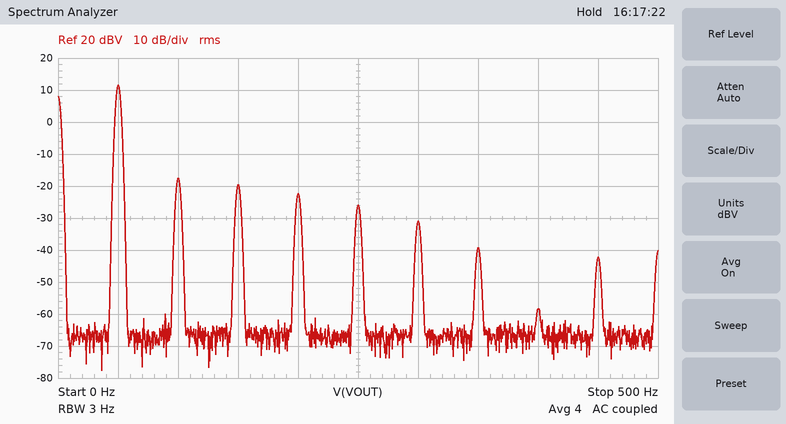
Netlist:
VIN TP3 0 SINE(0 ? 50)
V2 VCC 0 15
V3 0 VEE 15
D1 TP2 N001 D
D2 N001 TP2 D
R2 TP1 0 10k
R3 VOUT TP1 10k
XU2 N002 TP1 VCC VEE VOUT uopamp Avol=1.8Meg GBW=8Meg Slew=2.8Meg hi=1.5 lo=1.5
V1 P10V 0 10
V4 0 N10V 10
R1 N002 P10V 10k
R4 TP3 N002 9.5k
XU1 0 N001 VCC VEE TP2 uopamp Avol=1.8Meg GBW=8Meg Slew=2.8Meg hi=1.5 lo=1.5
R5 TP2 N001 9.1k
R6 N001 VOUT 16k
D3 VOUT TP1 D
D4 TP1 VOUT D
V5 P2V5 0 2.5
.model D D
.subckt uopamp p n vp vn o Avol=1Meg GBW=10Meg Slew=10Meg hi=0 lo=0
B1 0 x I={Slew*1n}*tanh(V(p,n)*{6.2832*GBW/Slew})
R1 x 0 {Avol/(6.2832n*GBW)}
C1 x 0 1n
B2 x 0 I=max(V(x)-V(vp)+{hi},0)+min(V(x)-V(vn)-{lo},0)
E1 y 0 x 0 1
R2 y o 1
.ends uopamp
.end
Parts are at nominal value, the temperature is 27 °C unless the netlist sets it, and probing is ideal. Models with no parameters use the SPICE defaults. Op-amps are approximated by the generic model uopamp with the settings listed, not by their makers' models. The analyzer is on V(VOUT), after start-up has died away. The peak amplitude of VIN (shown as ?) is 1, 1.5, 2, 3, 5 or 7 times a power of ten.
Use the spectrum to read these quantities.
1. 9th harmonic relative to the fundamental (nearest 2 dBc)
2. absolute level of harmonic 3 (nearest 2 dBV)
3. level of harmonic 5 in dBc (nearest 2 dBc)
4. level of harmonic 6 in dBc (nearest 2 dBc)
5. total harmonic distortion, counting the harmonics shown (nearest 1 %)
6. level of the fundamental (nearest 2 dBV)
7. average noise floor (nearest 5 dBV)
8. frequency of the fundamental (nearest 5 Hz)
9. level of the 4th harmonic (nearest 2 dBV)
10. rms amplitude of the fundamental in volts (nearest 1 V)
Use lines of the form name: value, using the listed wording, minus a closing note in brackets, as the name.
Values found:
9th harmonic relative to the fundamental: -54 dBc
absolute level of harmonic 3: -20 dBV
level of harmonic 5 in dBc: -38 dBc
level of harmonic 6 in dBc: -42 dBc
total harmonic distortion, counting the harmonics shown: 5 %
level of the fundamental: 12 dBV
average noise floor: -65 dBV
frequency of the fundamental: 50 Hz
level of the 4th harmonic: -22 dBV
rms amplitude of the fundamental in volts: 4 V
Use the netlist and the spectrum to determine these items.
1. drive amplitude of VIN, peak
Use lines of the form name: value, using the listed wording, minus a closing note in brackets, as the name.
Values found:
drive amplitude of VIN, peak: 10 V
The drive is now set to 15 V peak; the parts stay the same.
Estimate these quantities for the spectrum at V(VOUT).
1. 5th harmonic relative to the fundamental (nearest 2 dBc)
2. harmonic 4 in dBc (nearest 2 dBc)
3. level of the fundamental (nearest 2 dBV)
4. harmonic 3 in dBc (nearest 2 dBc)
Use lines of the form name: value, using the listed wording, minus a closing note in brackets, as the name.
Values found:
5th harmonic relative to the fundamental: -36 dBc
harmonic 4 in dBc: -42 dBc
level of the fundamental: 16 dBV
harmonic 3 in dBc: -38 dBc
